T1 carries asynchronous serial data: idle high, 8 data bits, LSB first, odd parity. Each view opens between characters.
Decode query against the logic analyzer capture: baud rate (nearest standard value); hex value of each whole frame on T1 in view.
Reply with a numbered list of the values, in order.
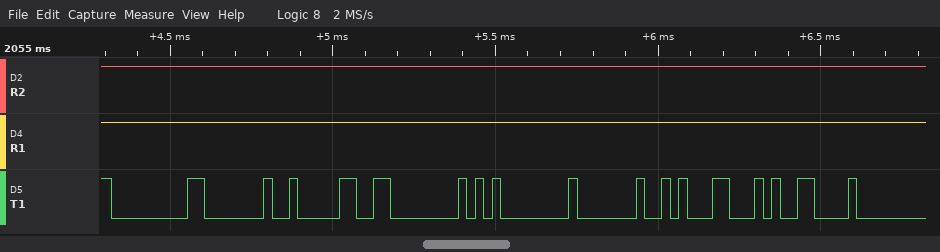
1. 38400 baud
2. 00, 40, 30, 80, 01, 40, 31, 19
